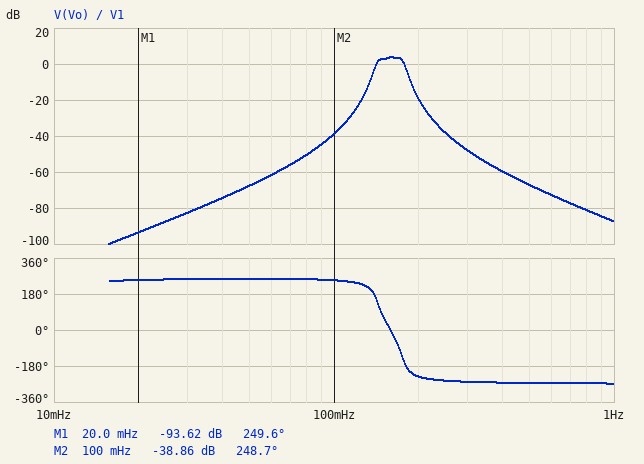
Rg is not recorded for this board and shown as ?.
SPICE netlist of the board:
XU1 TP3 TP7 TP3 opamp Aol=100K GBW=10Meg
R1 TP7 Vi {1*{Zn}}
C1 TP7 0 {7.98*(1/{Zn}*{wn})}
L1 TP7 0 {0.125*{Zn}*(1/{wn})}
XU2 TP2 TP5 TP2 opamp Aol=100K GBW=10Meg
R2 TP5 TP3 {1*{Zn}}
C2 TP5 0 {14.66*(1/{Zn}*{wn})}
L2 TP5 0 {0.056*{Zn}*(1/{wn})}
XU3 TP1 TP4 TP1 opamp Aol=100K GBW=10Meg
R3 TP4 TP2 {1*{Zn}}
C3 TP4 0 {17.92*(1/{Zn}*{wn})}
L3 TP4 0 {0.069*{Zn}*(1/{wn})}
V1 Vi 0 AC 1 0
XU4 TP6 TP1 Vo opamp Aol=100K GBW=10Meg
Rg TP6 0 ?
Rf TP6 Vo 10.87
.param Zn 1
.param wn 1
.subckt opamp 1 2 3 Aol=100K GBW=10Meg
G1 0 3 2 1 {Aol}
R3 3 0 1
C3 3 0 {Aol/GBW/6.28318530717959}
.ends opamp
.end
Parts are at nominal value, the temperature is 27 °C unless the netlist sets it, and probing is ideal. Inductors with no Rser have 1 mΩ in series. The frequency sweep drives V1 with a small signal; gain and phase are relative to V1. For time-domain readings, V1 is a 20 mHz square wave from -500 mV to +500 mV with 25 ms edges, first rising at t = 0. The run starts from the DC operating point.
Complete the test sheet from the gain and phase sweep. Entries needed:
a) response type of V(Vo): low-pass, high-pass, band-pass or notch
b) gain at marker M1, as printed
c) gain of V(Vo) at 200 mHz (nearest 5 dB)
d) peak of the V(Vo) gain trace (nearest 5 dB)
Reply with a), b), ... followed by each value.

a) band-pass
b) -93.62 dB
c) -20 dB
d) 5 dB
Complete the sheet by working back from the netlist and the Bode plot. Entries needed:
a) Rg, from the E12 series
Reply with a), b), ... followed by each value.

a) 0.56 Ω
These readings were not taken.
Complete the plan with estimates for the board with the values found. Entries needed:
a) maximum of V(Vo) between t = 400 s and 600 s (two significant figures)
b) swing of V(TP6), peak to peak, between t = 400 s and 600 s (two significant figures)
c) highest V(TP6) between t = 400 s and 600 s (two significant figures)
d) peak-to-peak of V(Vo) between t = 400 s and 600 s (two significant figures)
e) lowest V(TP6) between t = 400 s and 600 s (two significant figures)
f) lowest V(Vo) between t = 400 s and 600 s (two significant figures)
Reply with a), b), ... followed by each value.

a) 130 mV
b) 13 mV
c) 6.3 mV
d) 260 mV
e) -6.3 mV
f) -130 mV
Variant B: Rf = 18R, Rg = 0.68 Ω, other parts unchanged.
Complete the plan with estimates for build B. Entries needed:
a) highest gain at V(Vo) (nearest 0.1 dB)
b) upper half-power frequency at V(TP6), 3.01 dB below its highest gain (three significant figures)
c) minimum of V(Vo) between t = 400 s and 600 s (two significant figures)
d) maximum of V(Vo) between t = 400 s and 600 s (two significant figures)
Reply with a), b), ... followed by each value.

a) 6.3 dB
b) 178 mHz
c) -170 mV
d) 170 mV
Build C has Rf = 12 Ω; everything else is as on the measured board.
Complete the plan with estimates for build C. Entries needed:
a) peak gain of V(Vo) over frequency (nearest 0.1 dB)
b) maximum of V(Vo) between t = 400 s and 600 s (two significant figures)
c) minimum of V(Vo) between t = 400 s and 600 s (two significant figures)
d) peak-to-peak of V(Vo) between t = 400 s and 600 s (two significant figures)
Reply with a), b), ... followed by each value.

a) 4.5 dB
b) 140 mV
c) -140 mV
d) 280 mV
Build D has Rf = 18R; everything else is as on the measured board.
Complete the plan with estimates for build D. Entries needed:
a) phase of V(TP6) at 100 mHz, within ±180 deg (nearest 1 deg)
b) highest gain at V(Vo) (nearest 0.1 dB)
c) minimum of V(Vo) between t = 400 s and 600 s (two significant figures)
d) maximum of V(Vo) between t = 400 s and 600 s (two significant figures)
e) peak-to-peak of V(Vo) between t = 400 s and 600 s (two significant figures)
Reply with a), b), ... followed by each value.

a) -111 deg
b) 7.9 dB
c) -210 mV
d) 210 mV
e) 420 mV
